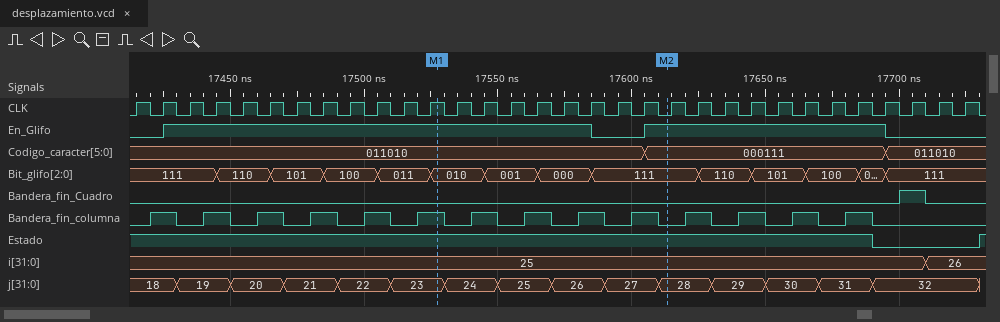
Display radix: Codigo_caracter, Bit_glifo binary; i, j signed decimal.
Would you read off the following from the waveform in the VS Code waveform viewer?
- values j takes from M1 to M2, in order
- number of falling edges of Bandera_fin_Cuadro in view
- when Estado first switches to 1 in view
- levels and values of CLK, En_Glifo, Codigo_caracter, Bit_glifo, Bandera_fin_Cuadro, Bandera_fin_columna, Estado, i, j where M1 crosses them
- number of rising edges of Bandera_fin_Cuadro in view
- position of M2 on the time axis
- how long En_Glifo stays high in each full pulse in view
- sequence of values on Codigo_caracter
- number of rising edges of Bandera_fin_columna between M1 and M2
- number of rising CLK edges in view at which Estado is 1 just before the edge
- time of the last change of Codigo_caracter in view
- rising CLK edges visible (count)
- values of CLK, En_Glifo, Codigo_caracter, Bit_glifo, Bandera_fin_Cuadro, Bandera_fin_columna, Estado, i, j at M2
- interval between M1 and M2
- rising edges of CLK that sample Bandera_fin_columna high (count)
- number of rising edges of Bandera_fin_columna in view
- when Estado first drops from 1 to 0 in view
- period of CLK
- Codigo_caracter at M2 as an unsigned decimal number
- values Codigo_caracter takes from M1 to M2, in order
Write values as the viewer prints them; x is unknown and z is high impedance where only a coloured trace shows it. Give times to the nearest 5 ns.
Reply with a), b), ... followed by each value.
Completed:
a) 23, 24, 25, 26, 27, 28
b) 1
c) 17730 ns
d) CLK=1, En_Glifo=1, Codigo_caracter=011010, Bit_glifo=010, Bandera_fin_Cuadro=0, Bandera_fin_columna=1, Estado=1, i=25, j=23
e) 1
f) 17615 ns
g) 160 ns, 90 ns
h) 011010, 000111, 011010
i) 4
j) 28
k) 17695 ns
l) 32
m) CLK=0, En_Glifo=1, Codigo_caracter=000111, Bit_glifo=111, Bandera_fin_Cuadro=0, Bandera_fin_columna=0, Estado=1, i=25, j=28
n) 85 ns
o) 14
p) 14
q) 17690 ns
r) 10 ns
s) 7
t) 011010, 000111
